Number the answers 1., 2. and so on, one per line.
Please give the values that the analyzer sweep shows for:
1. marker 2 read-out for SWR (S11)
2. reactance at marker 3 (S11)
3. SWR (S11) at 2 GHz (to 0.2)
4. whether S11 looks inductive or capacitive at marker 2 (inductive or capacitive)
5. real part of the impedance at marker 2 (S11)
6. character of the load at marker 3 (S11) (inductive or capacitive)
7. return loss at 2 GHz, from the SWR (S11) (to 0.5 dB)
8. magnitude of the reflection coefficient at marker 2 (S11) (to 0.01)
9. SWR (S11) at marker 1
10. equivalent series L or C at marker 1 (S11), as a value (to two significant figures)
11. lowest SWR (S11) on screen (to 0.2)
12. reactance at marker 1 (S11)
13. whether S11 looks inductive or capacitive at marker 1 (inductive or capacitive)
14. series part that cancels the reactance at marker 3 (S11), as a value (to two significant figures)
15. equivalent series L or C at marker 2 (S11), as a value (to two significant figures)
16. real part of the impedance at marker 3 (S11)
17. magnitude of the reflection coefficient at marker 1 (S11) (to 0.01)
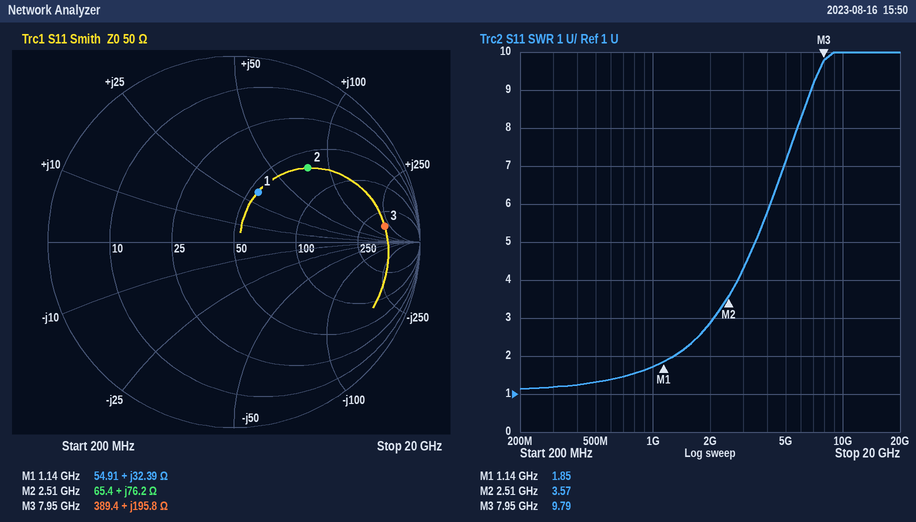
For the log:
1. 3.57
2. +195.8 Ω
3. 2.8
4. inductive
5. 65.4 Ω
6. inductive
7. 6.5 dB
8. 0.56
9. 1.85
10. 4.5 nH
11. 1.2
12. +32.39 Ω
13. inductive
14. 100 fF
15. 4.8 nH
16. 389.4 Ω
17. 0.30
